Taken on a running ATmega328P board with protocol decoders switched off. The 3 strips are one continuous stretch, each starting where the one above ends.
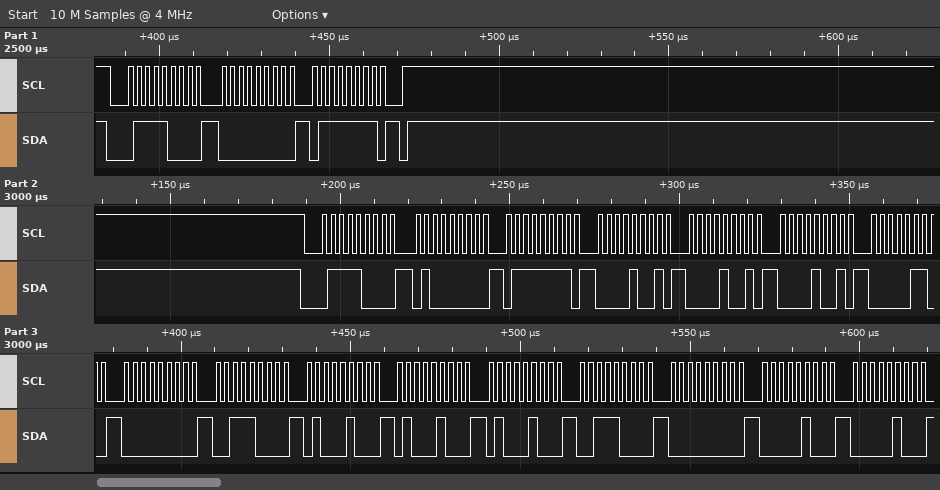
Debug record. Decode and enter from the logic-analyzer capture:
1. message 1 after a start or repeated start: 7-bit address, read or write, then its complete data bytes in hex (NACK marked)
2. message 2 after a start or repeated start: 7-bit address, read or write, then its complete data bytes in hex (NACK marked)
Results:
0x3C write: 00 7F
0x3C write: 40 7F 09 09 09 06 00 38 44 44 44 38 00 04 04
